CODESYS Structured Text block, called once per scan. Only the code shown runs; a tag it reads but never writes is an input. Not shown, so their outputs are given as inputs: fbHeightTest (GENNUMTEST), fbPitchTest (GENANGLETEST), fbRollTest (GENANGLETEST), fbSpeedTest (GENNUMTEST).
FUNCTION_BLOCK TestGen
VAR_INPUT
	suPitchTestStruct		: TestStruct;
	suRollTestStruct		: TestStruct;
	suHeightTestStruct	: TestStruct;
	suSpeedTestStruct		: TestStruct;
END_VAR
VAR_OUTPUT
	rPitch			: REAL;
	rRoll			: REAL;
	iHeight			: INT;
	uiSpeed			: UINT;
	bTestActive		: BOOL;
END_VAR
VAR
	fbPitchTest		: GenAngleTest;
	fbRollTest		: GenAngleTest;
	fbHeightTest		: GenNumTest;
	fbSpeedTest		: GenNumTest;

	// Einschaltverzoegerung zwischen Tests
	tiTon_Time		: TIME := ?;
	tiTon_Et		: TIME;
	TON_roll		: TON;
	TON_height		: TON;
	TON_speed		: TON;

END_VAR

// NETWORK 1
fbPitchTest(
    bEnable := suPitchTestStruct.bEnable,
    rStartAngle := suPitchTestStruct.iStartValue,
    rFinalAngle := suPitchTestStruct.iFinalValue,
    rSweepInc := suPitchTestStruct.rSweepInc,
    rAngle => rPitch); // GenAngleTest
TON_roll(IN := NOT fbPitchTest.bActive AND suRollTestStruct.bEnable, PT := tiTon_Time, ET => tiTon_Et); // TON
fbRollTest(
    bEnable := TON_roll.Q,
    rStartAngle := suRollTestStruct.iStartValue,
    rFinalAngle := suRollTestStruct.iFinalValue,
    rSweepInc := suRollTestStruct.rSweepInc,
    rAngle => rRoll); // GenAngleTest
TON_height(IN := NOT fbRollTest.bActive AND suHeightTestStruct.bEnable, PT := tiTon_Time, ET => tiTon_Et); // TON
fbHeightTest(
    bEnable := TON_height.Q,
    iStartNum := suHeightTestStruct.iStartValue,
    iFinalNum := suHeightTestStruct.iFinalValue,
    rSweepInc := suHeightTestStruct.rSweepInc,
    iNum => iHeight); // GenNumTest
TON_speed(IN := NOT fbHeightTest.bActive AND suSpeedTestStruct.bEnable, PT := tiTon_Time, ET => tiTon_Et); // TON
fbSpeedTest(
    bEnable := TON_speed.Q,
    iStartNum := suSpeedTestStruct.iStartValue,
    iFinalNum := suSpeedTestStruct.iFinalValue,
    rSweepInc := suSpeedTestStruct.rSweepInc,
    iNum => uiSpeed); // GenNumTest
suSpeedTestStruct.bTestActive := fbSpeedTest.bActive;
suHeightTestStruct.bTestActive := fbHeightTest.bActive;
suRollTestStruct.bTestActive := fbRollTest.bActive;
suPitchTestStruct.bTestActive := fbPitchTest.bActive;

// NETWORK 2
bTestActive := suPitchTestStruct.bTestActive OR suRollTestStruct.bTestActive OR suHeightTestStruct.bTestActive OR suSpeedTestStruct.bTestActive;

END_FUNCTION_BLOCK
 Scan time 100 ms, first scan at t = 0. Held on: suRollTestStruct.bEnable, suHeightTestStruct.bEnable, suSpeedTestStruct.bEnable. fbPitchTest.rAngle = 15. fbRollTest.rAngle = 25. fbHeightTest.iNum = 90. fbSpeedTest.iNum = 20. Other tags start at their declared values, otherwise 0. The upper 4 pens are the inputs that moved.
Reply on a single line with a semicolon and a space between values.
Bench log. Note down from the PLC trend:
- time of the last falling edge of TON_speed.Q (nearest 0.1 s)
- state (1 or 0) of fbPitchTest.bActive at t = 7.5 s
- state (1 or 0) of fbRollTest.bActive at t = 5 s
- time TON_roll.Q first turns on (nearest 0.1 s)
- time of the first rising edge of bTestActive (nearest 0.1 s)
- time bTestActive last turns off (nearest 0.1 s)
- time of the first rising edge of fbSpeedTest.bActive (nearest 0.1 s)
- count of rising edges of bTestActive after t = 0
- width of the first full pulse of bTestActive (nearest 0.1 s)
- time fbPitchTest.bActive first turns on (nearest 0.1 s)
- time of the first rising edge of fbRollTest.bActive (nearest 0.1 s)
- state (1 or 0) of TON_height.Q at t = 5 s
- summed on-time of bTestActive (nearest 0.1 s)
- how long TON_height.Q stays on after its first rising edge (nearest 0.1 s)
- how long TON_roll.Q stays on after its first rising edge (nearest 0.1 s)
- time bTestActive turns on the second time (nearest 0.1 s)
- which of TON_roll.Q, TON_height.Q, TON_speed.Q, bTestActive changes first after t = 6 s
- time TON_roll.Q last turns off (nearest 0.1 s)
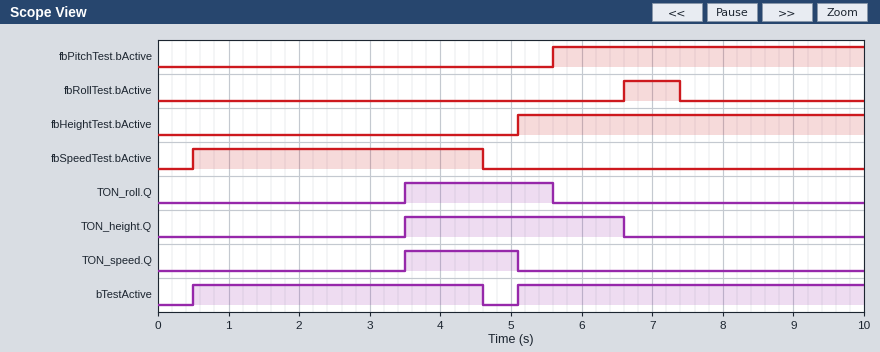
5.1 s; 1; 0; 3.5 s; 0.5 s; 4.6 s; 0.5 s; 2; 4.1 s; 5.6 s; 6.6 s; 1; 9.0 s; 3.1 s; 2.1 s; 5.1 s; TON_height.Q; 5.6 s
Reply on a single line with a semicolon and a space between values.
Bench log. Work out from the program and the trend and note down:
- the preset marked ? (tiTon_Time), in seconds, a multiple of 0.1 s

3.5 s
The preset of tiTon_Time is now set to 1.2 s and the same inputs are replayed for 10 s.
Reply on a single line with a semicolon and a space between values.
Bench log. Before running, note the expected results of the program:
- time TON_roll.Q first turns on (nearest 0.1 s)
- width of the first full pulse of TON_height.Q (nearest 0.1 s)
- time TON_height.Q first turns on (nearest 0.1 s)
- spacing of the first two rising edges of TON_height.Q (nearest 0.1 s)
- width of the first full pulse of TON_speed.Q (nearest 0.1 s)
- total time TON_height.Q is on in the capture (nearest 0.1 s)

1.2 s; 5.4 s; 1.2 s; 7.4 s; 3.9 s; 6.8 s
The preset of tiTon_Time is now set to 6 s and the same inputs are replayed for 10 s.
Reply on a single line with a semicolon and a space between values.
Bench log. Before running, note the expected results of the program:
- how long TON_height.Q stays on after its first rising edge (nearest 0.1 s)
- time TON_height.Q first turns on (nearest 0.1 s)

0.6 s; 6.0 s
